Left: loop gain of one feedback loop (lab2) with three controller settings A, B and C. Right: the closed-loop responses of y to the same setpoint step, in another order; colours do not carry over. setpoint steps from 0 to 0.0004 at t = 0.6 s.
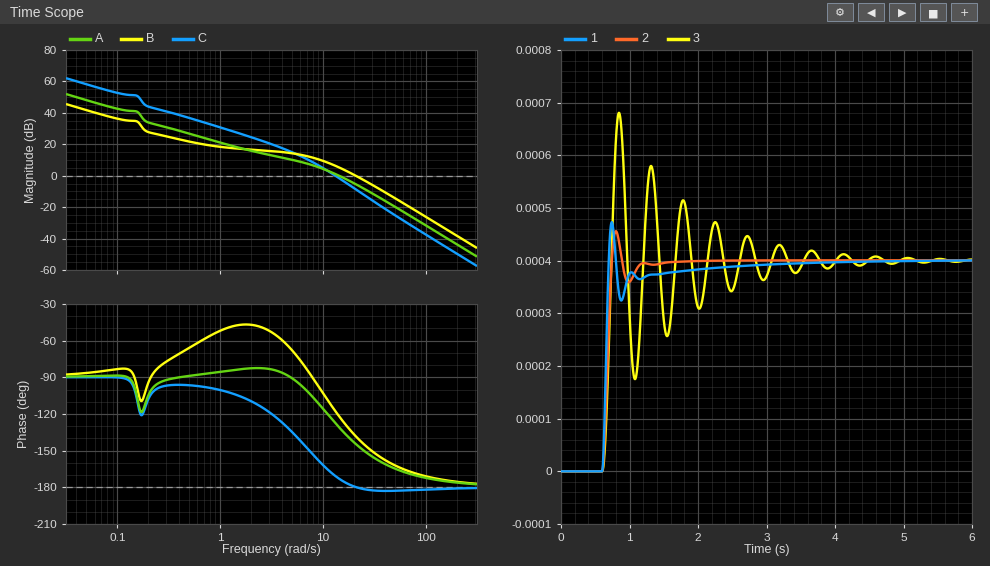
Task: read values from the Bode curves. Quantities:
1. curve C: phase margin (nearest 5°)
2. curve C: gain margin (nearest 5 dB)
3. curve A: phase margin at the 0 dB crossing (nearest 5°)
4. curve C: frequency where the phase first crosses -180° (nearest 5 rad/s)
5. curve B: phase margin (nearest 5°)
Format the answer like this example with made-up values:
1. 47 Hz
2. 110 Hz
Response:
1. 10°
2. 10 dB
3. 50°
4. 20 rad/s
5. 40°
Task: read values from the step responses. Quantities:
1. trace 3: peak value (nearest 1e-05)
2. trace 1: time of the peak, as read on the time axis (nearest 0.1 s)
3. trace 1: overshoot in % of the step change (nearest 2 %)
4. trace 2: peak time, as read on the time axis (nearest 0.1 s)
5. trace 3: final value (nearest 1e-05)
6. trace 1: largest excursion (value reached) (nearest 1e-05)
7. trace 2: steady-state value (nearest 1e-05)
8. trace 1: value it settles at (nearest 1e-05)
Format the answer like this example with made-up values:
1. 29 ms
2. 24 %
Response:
1. 0.00068
2. 0.7 s
3. 18 %
4. 0.8 s
5. 0.00040
6. 0.00047
7. 0.00040
8. 0.00040
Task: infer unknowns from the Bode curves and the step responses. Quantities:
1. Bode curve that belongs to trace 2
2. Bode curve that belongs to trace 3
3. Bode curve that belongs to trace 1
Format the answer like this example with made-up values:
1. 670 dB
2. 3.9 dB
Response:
1. A
2. C
3. B
